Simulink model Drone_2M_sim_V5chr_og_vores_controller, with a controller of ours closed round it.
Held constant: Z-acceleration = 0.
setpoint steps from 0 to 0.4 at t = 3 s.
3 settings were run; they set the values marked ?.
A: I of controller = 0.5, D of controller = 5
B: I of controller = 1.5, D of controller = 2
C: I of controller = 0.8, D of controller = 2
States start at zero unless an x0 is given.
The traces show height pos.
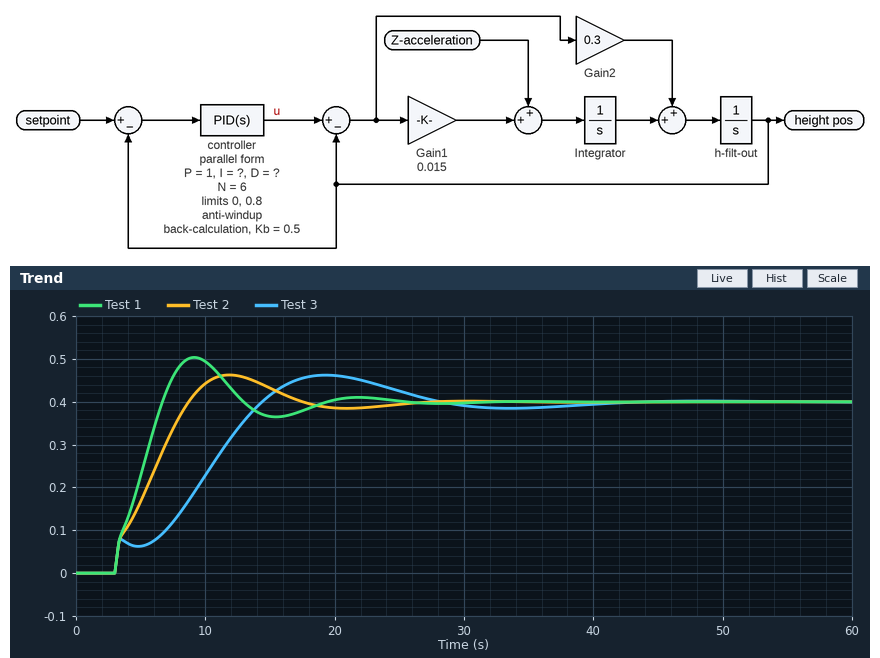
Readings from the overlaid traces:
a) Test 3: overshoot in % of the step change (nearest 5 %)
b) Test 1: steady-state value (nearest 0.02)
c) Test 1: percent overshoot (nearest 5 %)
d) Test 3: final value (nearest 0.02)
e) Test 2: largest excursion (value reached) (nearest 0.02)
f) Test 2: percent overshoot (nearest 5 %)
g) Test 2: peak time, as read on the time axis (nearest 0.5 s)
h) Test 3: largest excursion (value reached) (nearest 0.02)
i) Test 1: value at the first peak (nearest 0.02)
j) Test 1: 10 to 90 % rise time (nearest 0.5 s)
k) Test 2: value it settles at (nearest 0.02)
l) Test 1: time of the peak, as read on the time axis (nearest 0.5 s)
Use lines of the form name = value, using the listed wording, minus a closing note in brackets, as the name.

Test 3: overshoot in % of the step change = 15 %
Test 1: steady-state value = 0.40
Test 1: percent overshoot = 25 %
Test 3: final value = 0.40
Test 2: largest excursion (value reached) = 0.46
Test 2: percent overshoot = 15 %
Test 2: peak time, as read on the time axis = 12.0 s
Test 3: largest excursion (value reached) = 0.46
Test 1: value at the first peak = 0.50
Test 1: 10 to 90 % rise time = 3.0 s
Test 2: value it settles at = 0.40
Test 1: time of the peak, as read on the time axis = 9.0 s
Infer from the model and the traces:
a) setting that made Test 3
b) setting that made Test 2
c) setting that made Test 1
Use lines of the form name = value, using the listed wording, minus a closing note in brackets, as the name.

setting that made Test 3 = A
setting that made Test 2 = C
setting that made Test 1 = B
